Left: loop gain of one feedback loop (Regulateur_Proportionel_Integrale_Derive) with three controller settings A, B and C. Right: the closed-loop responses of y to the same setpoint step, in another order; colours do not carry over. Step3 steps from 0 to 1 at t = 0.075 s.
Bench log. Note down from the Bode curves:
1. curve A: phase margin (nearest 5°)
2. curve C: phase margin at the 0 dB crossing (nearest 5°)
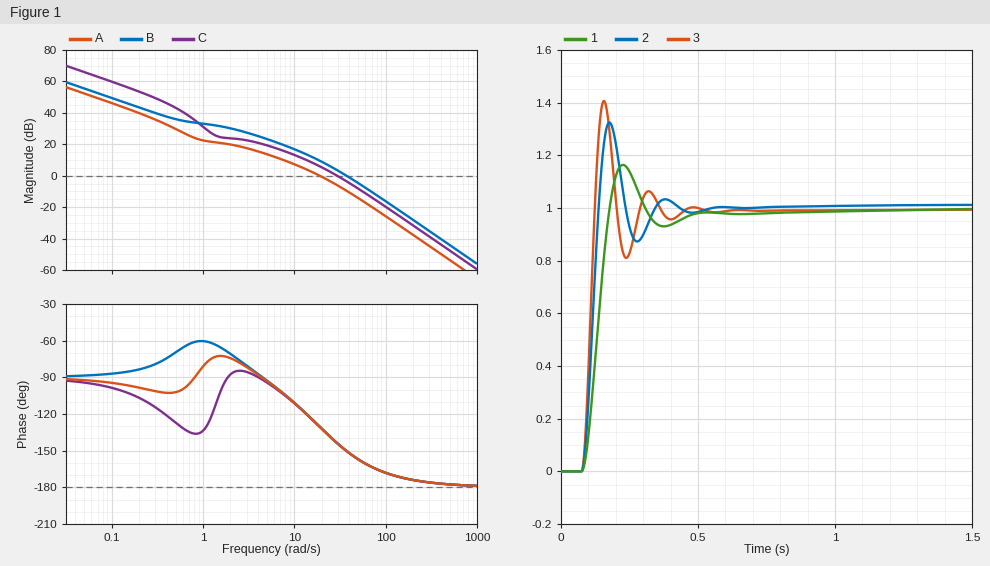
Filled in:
50°
35°
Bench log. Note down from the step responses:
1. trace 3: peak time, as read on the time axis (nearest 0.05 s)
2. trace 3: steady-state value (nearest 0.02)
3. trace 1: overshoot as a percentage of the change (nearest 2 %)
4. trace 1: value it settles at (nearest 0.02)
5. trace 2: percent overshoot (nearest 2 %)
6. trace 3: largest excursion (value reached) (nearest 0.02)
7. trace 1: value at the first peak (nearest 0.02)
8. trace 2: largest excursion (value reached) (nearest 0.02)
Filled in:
0.15 s
1.00
16 %
1.00
32 %
1.40
1.16
1.32
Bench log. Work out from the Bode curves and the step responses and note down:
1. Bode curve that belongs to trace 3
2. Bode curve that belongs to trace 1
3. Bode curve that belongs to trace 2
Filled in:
B
A
C
